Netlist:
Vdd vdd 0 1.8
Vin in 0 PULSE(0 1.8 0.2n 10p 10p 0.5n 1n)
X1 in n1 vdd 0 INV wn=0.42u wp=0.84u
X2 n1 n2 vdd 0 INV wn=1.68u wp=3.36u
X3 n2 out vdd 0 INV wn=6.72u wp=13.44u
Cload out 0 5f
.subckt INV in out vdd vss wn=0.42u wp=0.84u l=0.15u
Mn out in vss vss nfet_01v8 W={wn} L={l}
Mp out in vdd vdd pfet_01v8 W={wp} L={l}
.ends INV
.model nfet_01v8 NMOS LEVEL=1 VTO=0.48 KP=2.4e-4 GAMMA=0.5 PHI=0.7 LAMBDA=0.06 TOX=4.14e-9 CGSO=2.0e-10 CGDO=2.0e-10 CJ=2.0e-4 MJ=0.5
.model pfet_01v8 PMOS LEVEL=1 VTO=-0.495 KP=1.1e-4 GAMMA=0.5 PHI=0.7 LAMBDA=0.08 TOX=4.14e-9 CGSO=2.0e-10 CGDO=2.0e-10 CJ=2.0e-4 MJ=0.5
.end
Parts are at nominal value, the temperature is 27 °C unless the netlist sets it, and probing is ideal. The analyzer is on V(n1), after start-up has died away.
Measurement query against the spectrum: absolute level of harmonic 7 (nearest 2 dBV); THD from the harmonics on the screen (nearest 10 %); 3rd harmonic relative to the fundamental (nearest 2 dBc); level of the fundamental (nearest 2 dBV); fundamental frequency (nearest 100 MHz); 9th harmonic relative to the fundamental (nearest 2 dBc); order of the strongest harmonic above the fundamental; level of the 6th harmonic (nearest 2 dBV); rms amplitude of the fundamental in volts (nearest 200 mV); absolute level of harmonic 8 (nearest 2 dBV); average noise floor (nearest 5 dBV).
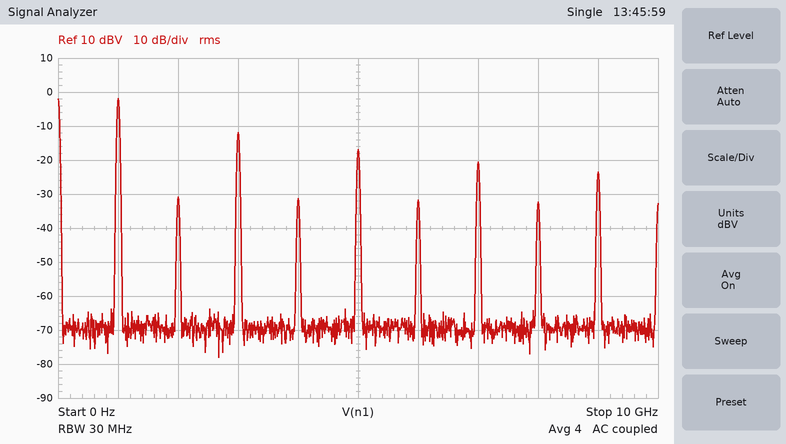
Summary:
-20 dBV
40 %
-10 dBc
-2 dBV
1.0 GHz
-22 dBc
3
-32 dBV
800 mV
-32 dBV
-70 dBV
